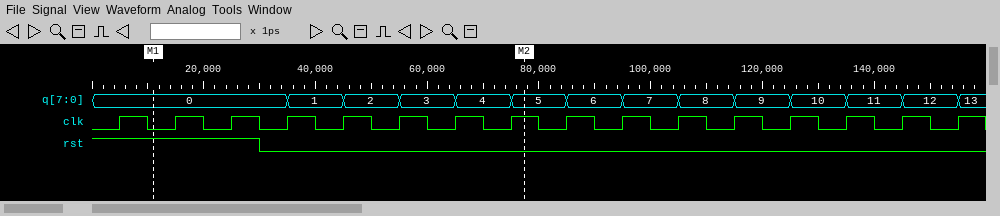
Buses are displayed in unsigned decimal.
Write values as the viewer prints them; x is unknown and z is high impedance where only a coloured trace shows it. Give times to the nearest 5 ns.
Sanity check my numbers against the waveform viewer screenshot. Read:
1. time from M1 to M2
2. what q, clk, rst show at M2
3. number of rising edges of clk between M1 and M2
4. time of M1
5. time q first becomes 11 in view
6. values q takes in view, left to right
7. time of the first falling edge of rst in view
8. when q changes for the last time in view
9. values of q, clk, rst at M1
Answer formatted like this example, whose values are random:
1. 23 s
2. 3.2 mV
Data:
1. 65 ns
2. q=5, clk=1, rst=0
3. 7
4. 10 ns
5. 135 ns
6. 0, 1, 2, 3, 4, 5, 6, 7, 8, 9, 10, 11, 12, 13
7. 30 ns
8. 155 ns
9. q=0, clk=0, rst=1
